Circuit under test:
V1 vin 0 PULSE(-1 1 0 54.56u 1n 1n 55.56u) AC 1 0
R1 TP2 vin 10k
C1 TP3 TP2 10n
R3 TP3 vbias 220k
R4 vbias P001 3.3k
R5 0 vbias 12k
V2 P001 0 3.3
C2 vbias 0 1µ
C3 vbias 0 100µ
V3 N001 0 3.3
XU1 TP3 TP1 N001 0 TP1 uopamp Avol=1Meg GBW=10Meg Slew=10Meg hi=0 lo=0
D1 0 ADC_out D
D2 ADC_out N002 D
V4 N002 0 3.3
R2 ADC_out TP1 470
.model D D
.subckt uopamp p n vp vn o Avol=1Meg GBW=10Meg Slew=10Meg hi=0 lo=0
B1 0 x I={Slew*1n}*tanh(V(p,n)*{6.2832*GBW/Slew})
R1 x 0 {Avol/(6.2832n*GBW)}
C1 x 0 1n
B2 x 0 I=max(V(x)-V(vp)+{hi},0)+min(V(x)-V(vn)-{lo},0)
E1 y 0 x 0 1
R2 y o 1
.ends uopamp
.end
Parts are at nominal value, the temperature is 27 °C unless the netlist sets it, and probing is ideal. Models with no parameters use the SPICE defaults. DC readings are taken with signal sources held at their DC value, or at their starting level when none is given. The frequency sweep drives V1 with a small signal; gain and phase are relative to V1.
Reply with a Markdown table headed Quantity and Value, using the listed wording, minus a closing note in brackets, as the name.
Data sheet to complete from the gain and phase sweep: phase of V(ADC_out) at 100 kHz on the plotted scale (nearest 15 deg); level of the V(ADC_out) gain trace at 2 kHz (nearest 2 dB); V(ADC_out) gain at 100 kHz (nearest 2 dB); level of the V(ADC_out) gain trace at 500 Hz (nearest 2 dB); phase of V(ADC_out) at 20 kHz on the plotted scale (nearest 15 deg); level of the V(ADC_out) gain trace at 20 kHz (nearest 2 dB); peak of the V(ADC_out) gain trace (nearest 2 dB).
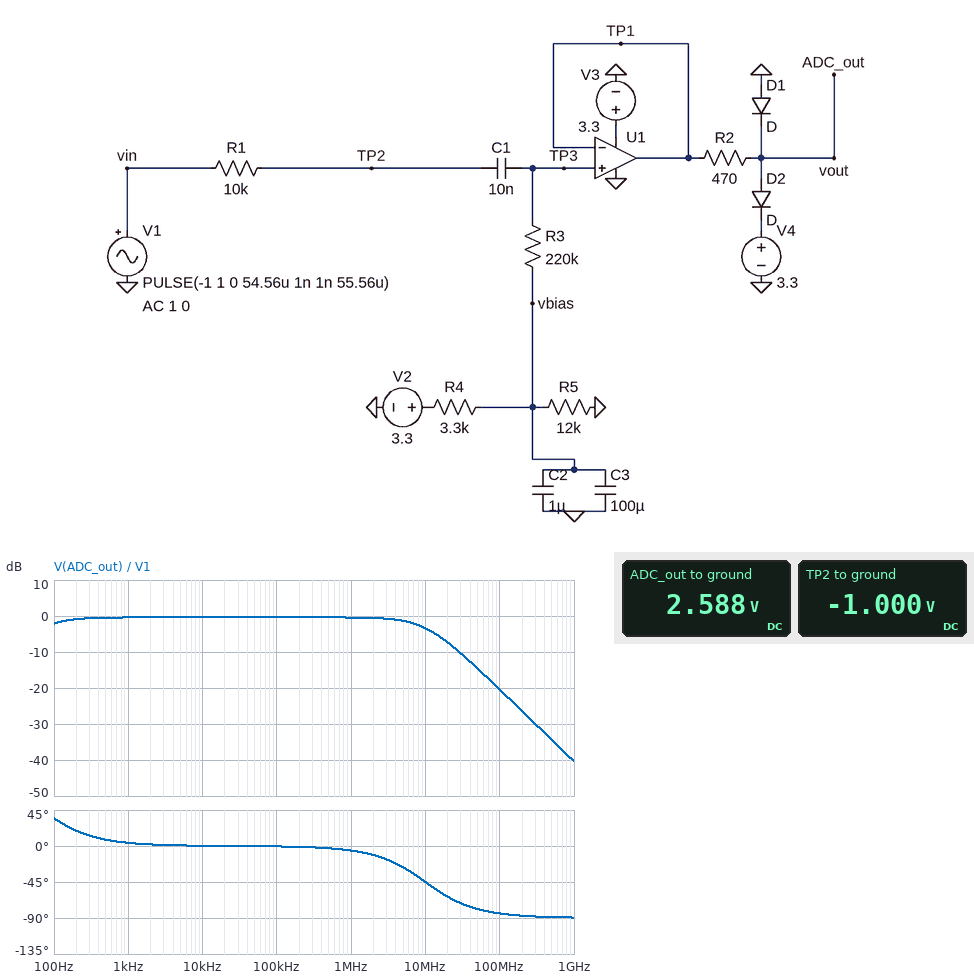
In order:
| Quantity | Value |
|---|---|
| phase of V(ADC_out) at 100 kHz on the plotted scale | 0 deg |
| level of the V(ADC_out) gain trace at 2 kHz | 0 dB |
| V(ADC_out) gain at 100 kHz | 0 dB |
| level of the V(ADC_out) gain trace at 500 Hz | 0 dB |
| phase of V(ADC_out) at 20 kHz on the plotted scale | 0 deg |
| level of the V(ADC_out) gain trace at 20 kHz | 0 dB |
| peak of the V(ADC_out) gain trace | 0 dB |
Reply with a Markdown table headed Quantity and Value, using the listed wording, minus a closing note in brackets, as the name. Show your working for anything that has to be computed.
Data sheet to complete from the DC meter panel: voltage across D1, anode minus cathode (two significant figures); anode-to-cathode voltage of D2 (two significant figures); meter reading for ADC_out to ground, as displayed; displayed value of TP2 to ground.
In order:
| Quantity | Value |
|---|---|
| voltage across D1, anode minus cathode | 0 V - 2.588 V = -2.6 V |
| anode-to-cathode voltage of D2 | 2.588 V - 3.3 V = -710 mV |
| meter reading for ADC_out to ground, as displayed | 2.588 V |
| displayed value of TP2 to ground | -1.000 V |
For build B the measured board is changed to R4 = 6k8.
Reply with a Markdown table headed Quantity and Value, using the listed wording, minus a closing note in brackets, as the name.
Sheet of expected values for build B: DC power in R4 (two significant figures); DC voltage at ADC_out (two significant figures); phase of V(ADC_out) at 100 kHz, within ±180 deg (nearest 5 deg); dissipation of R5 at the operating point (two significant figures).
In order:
| Quantity | Value |
|---|---|
| DC power in R4 | 210 µW |
| DC voltage at ADC_out | 2.1 V |
| phase of V(ADC_out) at 100 kHz, within ±180 deg | 0 deg |
| dissipation of R5 at the operating point | 370 µW |
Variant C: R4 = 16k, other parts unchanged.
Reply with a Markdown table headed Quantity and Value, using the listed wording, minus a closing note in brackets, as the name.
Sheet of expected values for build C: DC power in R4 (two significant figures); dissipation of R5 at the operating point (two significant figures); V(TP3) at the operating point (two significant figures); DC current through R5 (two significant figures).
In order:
| Quantity | Value |
|---|---|
| DC power in R4 | 220 µW |
| dissipation of R5 at the operating point | 170 µW |
| V(TP3) at the operating point | 1.4 V |
| DC current through R5 | 120 µA |
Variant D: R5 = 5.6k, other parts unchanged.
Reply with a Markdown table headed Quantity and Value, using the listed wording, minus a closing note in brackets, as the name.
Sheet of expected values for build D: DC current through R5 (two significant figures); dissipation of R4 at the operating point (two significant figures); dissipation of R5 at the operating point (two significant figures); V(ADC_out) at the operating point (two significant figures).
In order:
| Quantity | Value |
|---|---|
| DC current through R5 | 370 µA |
| dissipation of R4 at the operating point | 450 µW |
| dissipation of R5 at the operating point | 770 µW |
| V(ADC_out) at the operating point | 2.1 V |
